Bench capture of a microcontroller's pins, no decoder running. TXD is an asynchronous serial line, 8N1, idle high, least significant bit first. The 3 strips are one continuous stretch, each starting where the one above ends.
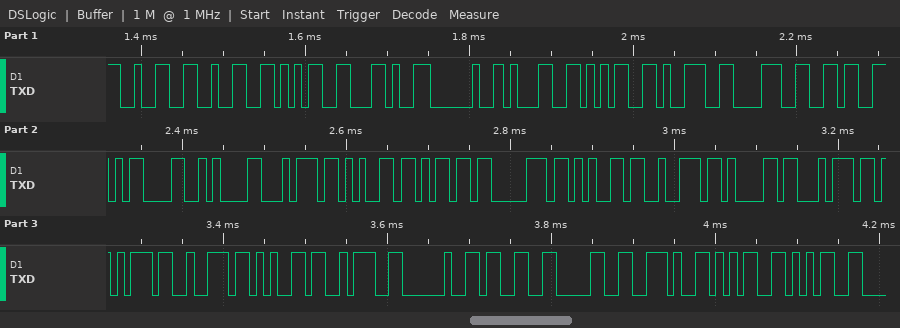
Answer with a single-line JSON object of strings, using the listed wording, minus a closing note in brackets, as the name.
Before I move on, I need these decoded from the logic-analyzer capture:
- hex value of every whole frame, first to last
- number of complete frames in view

{"hex value of every whole frame, first to last": "32 32 35 2C 20 31 35 39 38 36 0D 0A 74 65 6D 70 65 72 61 74 75 72 65 3A 20 33 30 2E 35 35", "number of complete frames in view": "30"}
